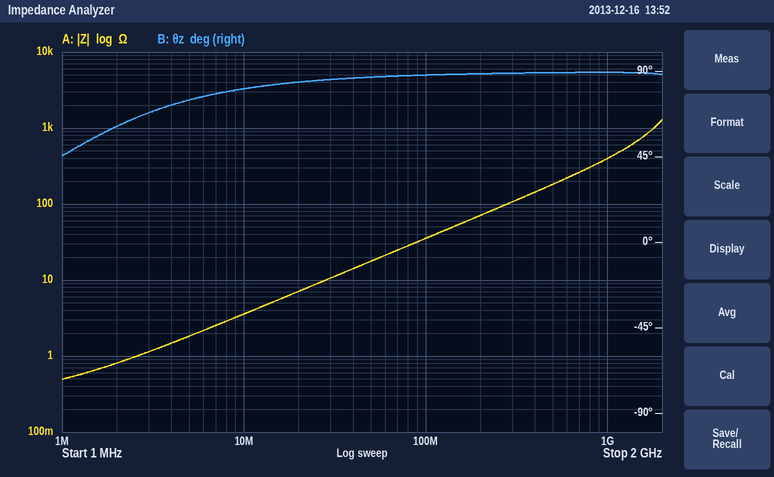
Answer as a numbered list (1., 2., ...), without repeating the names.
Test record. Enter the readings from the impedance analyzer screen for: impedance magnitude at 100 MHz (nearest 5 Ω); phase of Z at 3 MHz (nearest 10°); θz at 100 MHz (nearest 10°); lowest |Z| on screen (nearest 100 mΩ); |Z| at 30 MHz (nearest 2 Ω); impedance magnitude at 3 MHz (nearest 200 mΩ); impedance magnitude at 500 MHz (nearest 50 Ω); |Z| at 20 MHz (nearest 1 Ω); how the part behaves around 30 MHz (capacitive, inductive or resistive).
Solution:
1. 35 Ω
2. 70°
3. 90°
4. 500 mΩ
5. 10 Ω
6. 1.2 Ω
7. 200 Ω
8. 7 Ω
9. inductive
